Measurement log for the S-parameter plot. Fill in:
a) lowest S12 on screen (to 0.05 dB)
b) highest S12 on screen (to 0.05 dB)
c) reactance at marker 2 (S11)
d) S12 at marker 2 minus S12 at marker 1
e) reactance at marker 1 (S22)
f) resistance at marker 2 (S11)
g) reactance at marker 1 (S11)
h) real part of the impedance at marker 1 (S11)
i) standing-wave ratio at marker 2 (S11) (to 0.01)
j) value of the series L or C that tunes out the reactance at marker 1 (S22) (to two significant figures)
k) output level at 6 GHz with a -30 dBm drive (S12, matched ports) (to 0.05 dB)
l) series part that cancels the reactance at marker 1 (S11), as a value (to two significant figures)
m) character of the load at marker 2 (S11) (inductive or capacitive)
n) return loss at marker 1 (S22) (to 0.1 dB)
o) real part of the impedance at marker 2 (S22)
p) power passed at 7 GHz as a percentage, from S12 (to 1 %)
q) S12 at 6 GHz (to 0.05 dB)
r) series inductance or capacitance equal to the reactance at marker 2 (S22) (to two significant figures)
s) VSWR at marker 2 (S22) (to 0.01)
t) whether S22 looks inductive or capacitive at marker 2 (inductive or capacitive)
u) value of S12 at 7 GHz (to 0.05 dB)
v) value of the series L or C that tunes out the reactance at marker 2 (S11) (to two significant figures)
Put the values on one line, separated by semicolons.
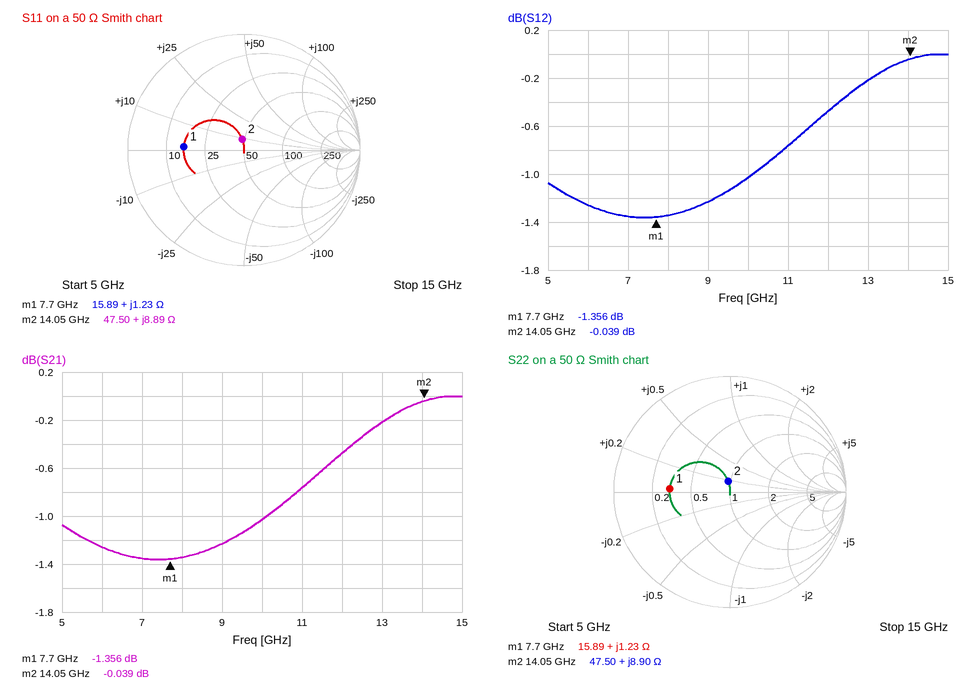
-1.35 dB; 0.00 dB; +8.89 Ω; 1.317 dB; +1.23 Ω; 47.50 Ω; +1.23 Ω; 15.89 Ω; 1.21; 17 pF; -31.25 dBm; 17 pF; inductive; 5.7 dB; 47.50 Ω; 73 %; -1.25 dB; 100 pH; 1.21; inductive; -1.35 dB; 1.3 pF
